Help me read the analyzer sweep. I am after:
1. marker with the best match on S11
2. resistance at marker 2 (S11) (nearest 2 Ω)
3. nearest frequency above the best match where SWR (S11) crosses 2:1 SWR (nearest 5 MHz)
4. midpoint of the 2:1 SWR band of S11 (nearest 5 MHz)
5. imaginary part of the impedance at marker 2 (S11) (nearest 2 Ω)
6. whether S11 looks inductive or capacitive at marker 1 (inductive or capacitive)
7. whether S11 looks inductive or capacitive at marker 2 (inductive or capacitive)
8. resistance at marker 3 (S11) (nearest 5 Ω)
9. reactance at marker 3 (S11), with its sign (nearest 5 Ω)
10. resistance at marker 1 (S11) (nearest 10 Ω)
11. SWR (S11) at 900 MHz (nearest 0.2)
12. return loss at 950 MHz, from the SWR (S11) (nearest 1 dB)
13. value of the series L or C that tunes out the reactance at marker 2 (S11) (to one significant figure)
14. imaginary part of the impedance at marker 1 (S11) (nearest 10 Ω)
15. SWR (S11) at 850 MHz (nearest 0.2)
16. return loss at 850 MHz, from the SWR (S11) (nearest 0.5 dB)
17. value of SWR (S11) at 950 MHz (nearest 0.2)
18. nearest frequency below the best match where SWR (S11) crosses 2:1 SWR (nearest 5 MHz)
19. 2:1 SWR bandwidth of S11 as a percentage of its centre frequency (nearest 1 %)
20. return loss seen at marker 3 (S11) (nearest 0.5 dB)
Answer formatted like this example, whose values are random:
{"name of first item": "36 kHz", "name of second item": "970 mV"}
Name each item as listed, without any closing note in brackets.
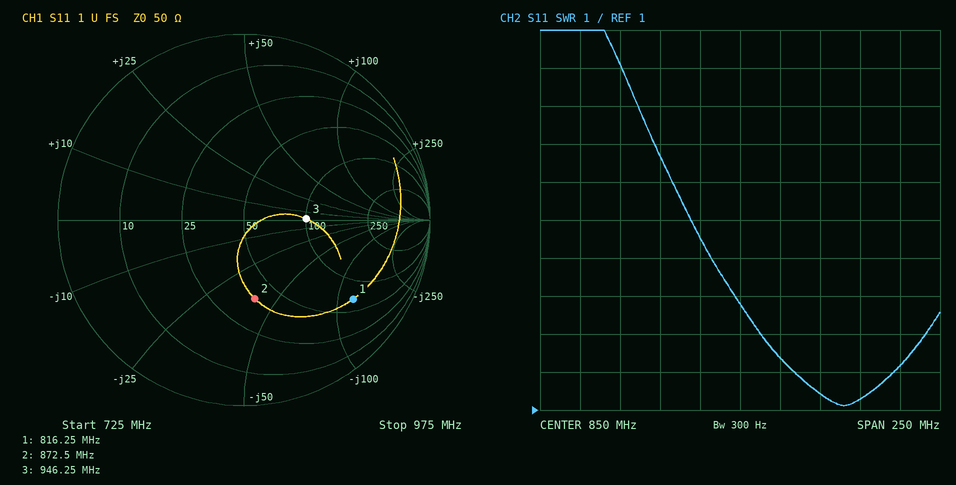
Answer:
{"marker with the best match on S11": "marker 3", "resistance at marker 2 (S11)": "38 Ω", "nearest frequency above the best match where SWR (S11) crosses 2:1 SWR": "945 MHz", "midpoint of the 2:1 SWR band of S11": "915 MHz", "imaginary part of the impedance at marker 2 (S11)": "-40 Ω", "whether S11 looks inductive or capacitive at marker 1": "capacitive", "whether S11 looks inductive or capacitive at marker 2": "capacitive", "resistance at marker 3 (S11)": "100 Ω", "reactance at marker 3 (S11), with its sign": "0 Ω", "resistance at marker 1 (S11)": "70 Ω", "SWR (S11) at 900 MHz": "1.4", "return loss at 950 MHz, from the SWR (S11)": "9 dB", "value of the series L or C that tunes out the reactance at marker 2 (S11)": "7 nH", "imaginary part of the impedance at marker 1 (S11)": "-120 Ω", "SWR (S11) at 850 MHz": "3.8", "return loss at 850 MHz, from the SWR (S11)": "4.5 dB", "value of SWR (S11) at 950 MHz": "2.2", "nearest frequency below the best match where SWR (S11) crosses 2:1 SWR": "885 MHz", "2:1 SWR bandwidth of S11 as a percentage of its centre frequency": "7 %", "return loss seen at marker 3 (S11)": "9.5 dB"}
